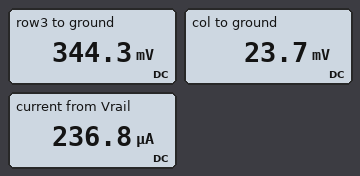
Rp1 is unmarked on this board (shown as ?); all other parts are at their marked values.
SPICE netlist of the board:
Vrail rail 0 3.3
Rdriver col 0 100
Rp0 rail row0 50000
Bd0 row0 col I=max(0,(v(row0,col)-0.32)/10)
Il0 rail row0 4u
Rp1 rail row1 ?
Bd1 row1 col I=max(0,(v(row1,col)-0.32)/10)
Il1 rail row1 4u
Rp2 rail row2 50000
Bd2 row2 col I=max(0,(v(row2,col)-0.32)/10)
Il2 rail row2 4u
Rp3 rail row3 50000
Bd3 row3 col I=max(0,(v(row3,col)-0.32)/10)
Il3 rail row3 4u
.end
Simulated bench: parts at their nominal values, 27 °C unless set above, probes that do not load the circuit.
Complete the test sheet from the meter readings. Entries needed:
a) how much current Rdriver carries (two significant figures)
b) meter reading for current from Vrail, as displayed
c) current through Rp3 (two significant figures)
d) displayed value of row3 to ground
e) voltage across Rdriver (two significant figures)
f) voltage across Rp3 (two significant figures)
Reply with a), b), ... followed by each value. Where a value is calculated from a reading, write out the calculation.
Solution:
a) (23.7 mV) / 100 Ω = 240 µA
b) 236.8 µA
c) (3.3 V - 344.3 mV) / 50 kΩ = 59 µA
d) 344.3 mV
e) 23.7 mV = 24 mV
f) 3.3 V - 344.3 mV = 3.0 V
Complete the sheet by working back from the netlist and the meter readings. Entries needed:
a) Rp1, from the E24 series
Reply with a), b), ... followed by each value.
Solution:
a) 68 kΩ
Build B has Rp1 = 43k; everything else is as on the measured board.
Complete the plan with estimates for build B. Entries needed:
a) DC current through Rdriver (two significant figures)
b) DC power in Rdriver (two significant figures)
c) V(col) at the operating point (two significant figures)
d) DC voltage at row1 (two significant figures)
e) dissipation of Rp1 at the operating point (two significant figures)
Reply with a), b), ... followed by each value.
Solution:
a) 260 µA
b) 6.9 µW
c) 26 mV
d) 350 mV
e) 200 µW
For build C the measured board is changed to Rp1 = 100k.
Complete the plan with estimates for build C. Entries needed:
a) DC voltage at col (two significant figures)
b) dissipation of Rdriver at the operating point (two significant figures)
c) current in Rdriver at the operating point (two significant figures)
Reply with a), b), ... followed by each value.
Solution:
a) 22 mV
b) 5.0 µW
c) 220 µA
